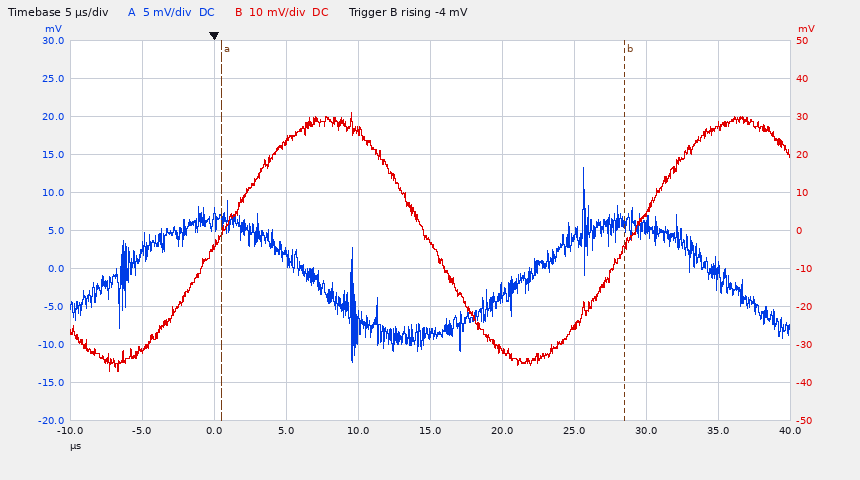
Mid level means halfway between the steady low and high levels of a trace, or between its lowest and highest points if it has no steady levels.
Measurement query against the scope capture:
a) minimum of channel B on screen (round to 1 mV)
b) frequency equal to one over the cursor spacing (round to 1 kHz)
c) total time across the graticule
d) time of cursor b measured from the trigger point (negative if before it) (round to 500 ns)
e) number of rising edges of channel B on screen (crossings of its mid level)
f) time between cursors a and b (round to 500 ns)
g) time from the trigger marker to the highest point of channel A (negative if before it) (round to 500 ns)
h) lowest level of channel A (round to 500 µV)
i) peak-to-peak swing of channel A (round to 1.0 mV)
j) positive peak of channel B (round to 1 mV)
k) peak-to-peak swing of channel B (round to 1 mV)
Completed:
-37 mV
36 kHz
50 µs
+28.5 µs
2
28.0 µs
+25.5 µs
-12.5 mV
26.0 mV
31 mV
68 mV
